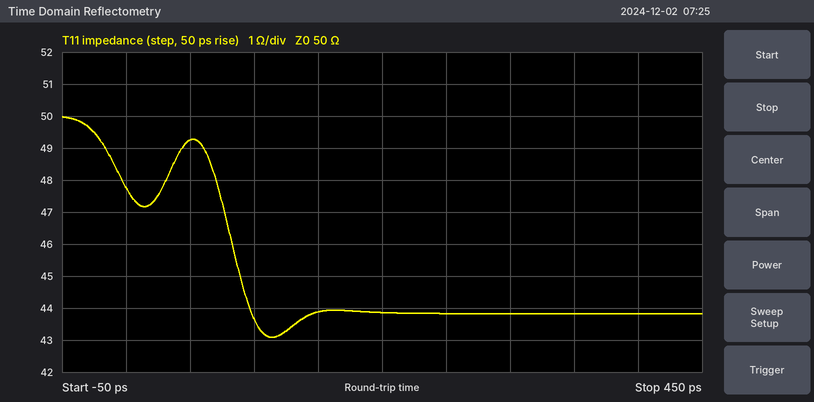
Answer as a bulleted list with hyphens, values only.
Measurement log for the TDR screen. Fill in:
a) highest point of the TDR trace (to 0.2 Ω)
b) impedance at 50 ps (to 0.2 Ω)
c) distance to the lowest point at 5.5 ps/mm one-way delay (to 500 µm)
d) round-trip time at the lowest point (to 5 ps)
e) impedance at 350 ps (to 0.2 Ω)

- 50.0 Ω
- 49.2 Ω
- 10.5 mm
- 115 ps
- 43.8 Ω
